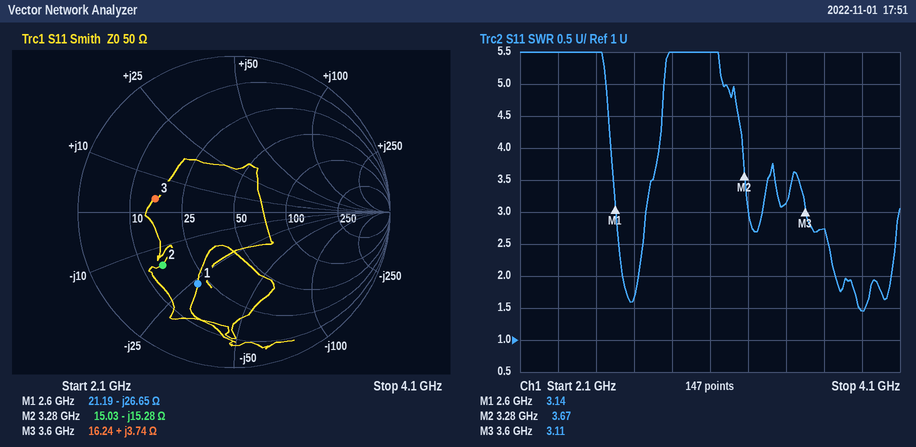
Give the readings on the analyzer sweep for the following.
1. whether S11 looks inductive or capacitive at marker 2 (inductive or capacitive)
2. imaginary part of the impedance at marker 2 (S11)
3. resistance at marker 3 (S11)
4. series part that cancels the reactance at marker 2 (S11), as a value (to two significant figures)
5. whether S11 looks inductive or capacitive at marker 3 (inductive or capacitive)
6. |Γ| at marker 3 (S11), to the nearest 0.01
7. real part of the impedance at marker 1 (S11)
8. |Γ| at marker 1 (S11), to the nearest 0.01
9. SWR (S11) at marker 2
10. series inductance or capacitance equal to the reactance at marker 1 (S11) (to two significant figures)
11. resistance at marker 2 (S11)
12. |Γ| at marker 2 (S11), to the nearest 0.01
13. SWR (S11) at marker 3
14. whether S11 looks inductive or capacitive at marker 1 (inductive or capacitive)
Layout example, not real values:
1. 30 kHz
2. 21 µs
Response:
1. capacitive
2. -15.28 Ω
3. 16.24 Ω
4. 740 pH
5. inductive
6. 0.51
7. 21.19 Ω
8. 0.52
9. 3.67
10. 2.3 pF
11. 15.03 Ω
12. 0.57
13. 3.11
14. capacitive
